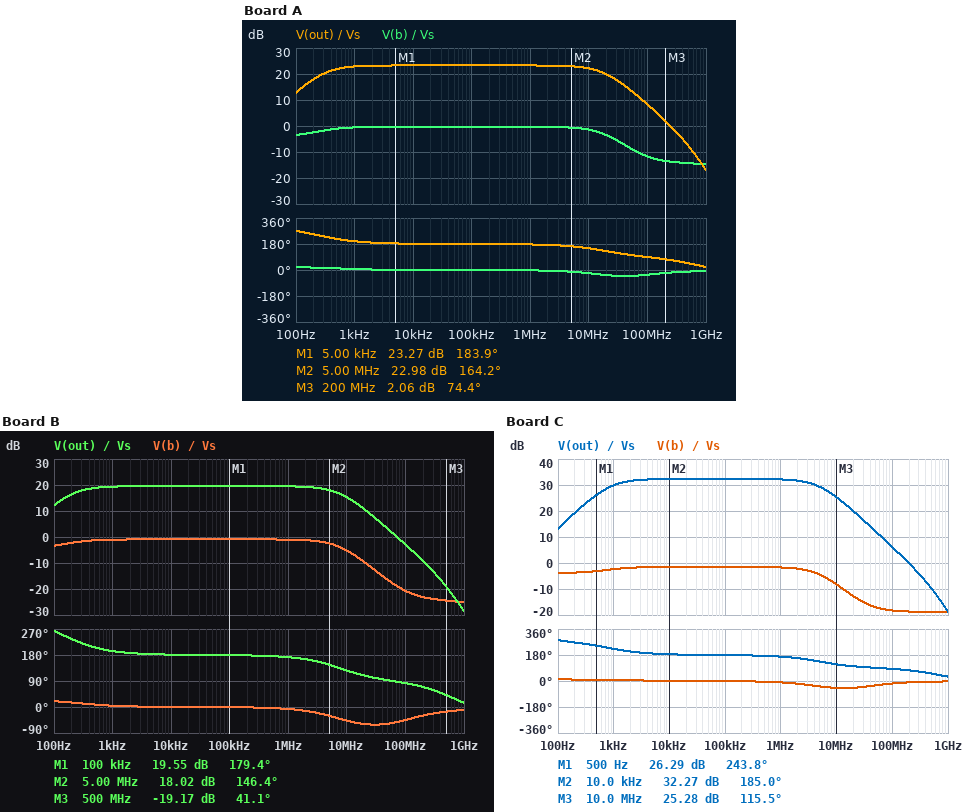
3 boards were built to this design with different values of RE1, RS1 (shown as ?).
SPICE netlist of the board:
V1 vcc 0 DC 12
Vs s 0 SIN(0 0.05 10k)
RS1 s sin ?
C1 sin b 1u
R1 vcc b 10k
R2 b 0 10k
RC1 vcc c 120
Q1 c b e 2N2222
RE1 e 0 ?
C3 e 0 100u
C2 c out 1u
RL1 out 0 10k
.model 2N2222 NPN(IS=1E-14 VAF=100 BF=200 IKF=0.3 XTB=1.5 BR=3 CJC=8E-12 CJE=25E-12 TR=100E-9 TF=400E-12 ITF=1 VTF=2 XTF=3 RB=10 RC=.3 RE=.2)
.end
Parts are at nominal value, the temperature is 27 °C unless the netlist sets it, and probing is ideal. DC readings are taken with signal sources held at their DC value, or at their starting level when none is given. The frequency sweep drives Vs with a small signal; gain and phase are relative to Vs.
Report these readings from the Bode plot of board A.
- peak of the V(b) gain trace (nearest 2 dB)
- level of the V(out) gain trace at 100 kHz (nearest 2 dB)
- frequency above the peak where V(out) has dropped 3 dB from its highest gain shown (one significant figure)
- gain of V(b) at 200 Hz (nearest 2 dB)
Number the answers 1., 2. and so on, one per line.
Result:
1. 0 dB
2. 24 dB
3. 20 MHz
4. -2 dB
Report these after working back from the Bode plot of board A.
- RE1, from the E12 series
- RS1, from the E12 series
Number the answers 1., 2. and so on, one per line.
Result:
1. 1.5 kΩ
2. 47 Ω
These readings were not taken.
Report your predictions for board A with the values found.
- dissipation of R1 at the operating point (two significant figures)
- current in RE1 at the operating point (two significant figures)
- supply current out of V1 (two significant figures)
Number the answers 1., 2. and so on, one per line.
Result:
1. 3.7 mW
2. 3.5 mA
3. 4.1 mA
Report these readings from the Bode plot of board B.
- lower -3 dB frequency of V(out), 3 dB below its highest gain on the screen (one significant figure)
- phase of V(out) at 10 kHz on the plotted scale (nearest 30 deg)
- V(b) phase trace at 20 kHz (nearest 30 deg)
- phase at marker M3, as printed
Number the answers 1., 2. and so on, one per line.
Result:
1. 200 Hz
2. 180 deg
3. 0 deg
4. 41.1 deg
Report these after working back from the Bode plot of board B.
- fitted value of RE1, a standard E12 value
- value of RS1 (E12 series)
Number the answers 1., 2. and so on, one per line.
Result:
1. 2.2 kΩ
2. 180 Ω
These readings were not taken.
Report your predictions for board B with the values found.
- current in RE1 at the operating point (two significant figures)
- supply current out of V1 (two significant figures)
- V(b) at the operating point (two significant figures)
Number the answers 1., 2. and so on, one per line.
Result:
1. 2.4 mA
2. 3.0 mA
3. 5.9 V
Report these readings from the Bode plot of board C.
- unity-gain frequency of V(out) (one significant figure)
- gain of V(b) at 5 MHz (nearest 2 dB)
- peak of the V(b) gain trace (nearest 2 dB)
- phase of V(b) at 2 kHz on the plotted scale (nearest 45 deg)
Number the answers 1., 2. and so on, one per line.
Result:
1. 200 MHz
2. -4 dB
3. -2 dB
4. 0 deg
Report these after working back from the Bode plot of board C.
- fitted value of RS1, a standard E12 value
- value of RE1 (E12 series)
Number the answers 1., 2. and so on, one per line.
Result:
1. 82 Ω
2. 390 Ω
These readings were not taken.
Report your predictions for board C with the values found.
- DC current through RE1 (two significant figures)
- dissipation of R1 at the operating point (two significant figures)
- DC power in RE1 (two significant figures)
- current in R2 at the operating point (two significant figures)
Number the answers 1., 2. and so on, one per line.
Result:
1. 13 mA
2. 4.0 mW
3. 63 mW
4. 570 µA
